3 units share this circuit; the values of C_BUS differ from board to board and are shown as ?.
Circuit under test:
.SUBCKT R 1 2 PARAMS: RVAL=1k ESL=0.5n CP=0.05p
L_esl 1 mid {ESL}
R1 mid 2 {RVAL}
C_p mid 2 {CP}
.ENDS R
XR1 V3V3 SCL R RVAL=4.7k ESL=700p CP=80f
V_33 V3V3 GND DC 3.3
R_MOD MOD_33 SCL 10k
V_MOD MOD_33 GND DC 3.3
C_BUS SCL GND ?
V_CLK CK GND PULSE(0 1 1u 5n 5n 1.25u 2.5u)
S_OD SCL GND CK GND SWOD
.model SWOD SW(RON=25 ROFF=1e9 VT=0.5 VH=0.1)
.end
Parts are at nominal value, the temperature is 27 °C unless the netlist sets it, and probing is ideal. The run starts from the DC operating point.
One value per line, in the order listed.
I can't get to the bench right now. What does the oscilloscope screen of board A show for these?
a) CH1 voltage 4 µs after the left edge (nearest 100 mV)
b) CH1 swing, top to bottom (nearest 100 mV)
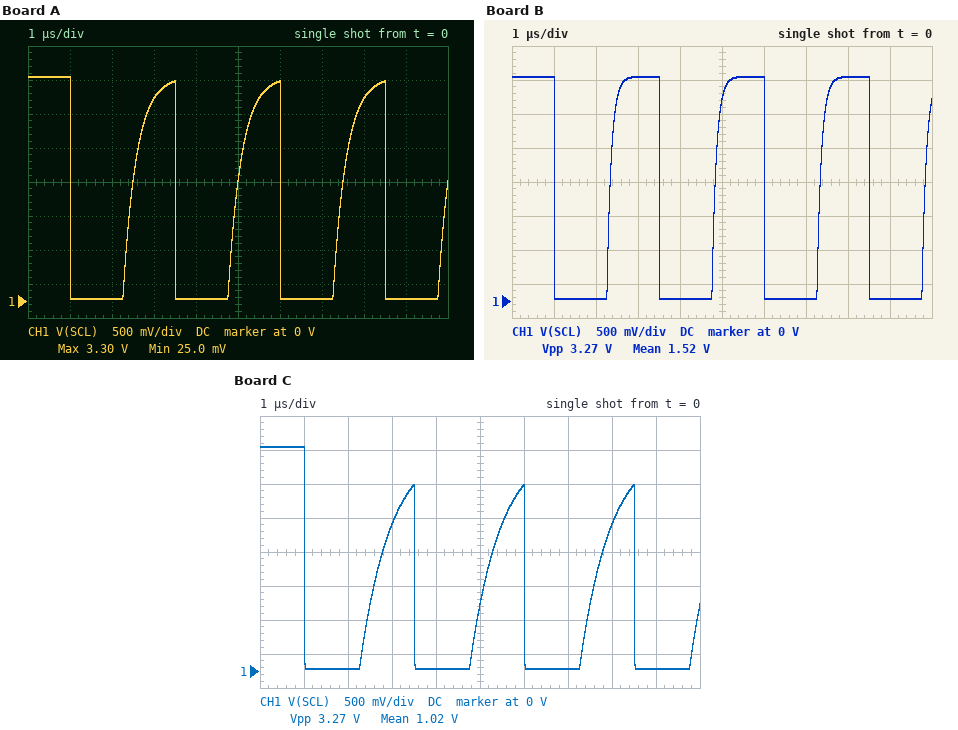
0 V
3.3 V
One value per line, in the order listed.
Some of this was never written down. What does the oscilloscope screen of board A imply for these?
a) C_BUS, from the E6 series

100 pF
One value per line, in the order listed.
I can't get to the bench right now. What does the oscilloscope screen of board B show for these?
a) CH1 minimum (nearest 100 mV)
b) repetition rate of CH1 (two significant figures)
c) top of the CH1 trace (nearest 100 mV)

0 V
400 kHz
3.3 V
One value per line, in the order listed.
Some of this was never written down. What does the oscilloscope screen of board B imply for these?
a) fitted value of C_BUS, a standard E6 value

33 pF
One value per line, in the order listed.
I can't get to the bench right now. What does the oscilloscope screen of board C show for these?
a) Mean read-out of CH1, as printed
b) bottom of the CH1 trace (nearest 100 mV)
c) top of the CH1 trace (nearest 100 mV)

1.02 V
0 V
3.3 V
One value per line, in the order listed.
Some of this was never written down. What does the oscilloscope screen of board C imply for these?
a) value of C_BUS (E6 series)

220 pF
